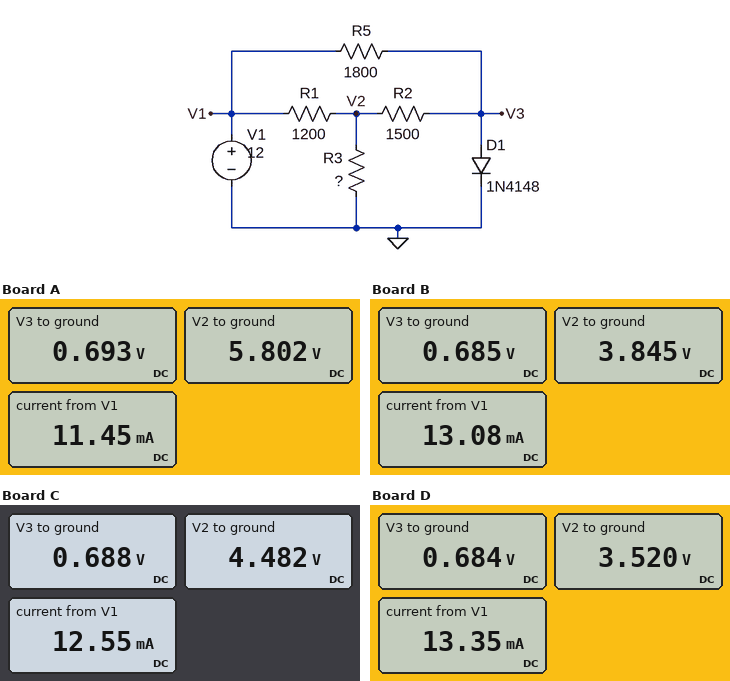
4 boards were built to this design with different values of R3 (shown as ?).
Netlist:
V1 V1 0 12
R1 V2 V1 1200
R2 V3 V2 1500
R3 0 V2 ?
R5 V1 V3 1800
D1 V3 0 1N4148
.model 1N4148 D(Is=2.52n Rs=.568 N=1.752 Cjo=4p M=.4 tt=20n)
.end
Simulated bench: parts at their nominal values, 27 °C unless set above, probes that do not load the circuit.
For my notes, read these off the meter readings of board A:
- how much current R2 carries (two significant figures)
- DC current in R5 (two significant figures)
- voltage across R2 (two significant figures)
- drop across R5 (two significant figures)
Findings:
3.4 mA
6.3 mA
5.1 V
11 V
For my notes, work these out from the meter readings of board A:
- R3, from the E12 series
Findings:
3.3 kΩ
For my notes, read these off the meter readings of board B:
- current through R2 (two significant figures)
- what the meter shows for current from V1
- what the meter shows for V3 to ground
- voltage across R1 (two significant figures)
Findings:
2.1 mA
13.08 mA
0.685 V
8.2 V
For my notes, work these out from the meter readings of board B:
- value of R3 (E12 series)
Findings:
820 Ω
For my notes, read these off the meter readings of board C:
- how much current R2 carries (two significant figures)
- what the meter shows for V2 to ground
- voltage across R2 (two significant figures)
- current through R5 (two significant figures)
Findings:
2.5 mA
4.482 V
3.8 V
6.3 mA
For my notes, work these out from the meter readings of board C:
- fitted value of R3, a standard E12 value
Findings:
1.2 kΩ
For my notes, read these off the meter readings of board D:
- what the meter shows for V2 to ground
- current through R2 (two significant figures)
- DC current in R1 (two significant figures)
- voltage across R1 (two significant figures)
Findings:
3.520 V
1.9 mA
7.1 mA
8.5 V
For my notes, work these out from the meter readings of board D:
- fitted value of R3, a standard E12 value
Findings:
680 Ω
